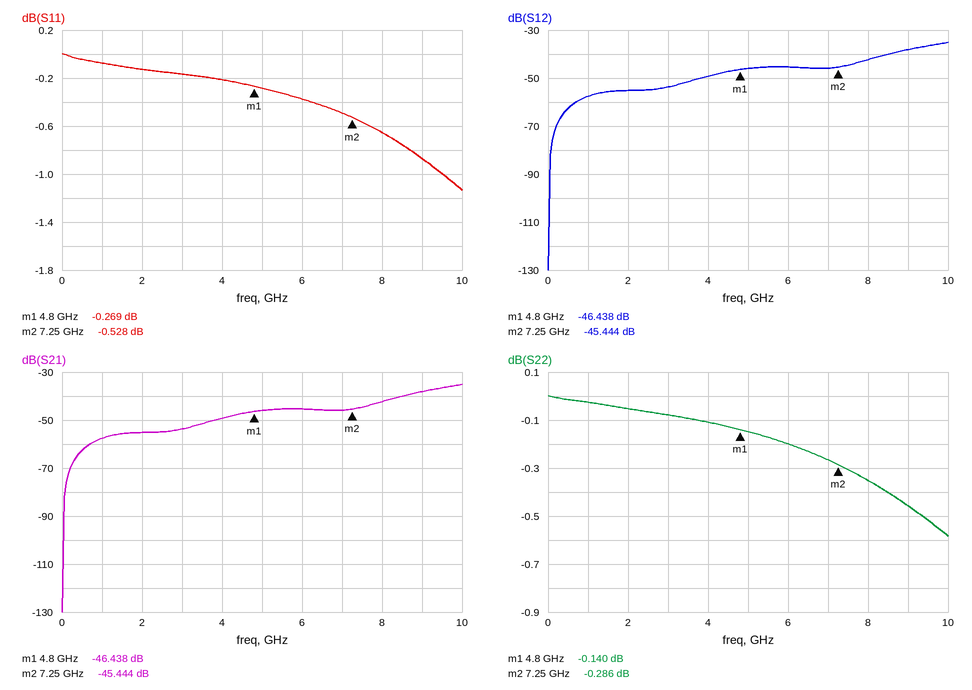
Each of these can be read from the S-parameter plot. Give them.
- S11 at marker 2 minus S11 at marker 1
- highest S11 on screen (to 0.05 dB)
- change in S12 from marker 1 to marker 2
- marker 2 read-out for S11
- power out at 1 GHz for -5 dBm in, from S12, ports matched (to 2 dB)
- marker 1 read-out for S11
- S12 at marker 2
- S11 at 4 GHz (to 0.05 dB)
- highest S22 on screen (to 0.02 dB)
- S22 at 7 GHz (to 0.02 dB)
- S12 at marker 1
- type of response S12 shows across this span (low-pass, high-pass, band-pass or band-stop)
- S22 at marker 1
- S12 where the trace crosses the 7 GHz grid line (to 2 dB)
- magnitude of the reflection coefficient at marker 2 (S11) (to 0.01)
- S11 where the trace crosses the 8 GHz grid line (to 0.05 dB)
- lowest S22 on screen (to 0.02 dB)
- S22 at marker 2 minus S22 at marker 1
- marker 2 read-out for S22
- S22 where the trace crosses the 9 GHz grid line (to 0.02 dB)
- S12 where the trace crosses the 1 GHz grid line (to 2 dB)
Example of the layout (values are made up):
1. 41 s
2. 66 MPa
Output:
1. -0.259 dB
2. 0.00 dB
3. 0.994 dB
4. -0.528 dB
5. -62 dBm
6. -0.269 dB
7. -45.444 dB
8. -0.20 dB
9. 0.00 dB
10. -0.26 dB
11. -46.438 dB
12. high-pass
13. -0.140 dB
14. -46 dB
15. 0.94
16. -0.65 dB
17. -0.58 dB
18. -0.146 dB
19. -0.286 dB
20. -0.46 dB
21. -58 dB
